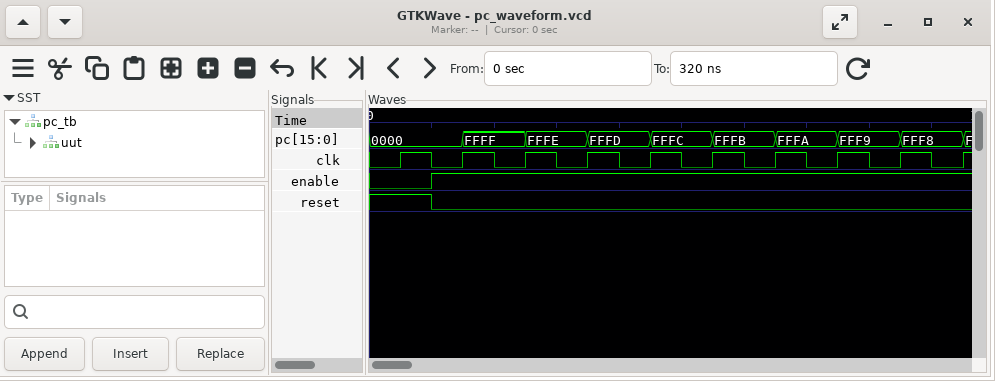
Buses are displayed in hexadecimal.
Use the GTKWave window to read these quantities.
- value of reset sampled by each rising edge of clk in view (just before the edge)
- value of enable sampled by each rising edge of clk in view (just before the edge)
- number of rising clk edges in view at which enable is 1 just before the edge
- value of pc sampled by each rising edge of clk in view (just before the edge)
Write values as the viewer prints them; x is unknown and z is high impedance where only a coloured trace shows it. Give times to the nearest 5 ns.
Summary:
1 0 0 0 0 0 0 0 0 0
0 1 1 1 1 1 1 1 1 1
9
0000, 0000, FFFF, FFFE, FFFD, FFFC, FFFB, FFFA, FFF9, FFF8
